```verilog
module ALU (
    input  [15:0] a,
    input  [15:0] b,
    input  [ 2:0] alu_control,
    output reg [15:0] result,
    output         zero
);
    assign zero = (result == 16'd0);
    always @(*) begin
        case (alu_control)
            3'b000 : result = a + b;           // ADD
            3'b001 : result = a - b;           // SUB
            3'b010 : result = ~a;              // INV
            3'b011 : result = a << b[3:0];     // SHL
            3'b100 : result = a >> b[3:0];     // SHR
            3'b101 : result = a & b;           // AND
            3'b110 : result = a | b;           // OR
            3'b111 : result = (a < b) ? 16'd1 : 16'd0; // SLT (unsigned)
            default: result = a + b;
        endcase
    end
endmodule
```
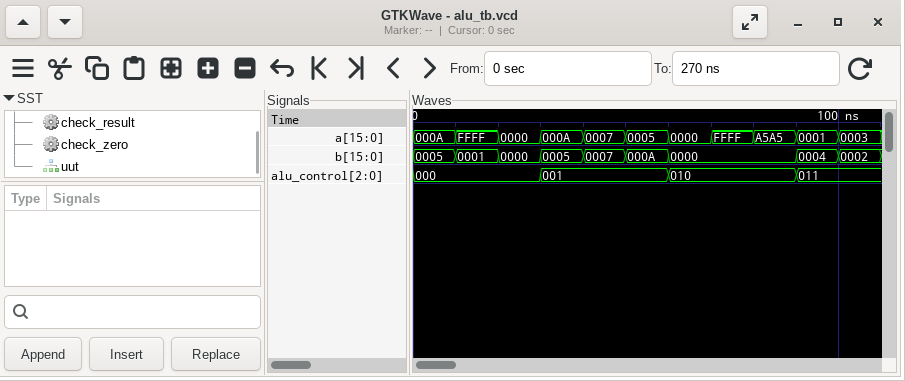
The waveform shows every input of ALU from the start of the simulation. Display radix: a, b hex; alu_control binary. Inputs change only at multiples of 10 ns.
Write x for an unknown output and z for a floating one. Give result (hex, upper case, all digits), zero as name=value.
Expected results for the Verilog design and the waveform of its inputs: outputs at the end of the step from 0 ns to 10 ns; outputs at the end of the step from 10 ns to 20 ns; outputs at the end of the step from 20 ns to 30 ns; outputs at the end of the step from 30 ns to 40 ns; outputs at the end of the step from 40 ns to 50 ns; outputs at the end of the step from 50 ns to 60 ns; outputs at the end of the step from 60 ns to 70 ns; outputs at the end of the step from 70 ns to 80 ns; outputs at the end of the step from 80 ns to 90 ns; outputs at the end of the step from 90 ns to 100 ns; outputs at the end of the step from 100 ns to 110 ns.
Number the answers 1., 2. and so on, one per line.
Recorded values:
1. result=000F, zero=0
2. result=0000, zero=1
3. result=0000, zero=1
4. result=0005, zero=0
5. result=0000, zero=1
6. result=FFFB, zero=0
7. result=FFFF, zero=0
8. result=0000, zero=1
9. result=5A5A, zero=0
10. result=0010, zero=0
11. result=000C, zero=0
